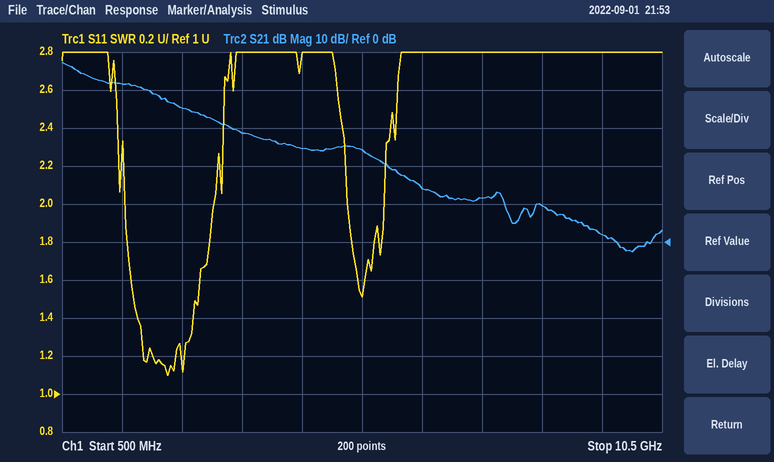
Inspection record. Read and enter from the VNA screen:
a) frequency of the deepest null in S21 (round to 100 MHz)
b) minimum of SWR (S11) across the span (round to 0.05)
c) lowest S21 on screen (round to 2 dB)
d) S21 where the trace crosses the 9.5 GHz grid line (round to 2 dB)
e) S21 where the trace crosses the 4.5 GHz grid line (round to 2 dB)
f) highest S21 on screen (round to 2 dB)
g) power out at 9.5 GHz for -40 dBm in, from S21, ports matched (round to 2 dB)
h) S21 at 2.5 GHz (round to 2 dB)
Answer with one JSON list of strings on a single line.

["10.0 GHz", "1.10", "-2 dB", "2 dB", "24 dB", "48 dB", "-38 dBm", "36 dB"]
